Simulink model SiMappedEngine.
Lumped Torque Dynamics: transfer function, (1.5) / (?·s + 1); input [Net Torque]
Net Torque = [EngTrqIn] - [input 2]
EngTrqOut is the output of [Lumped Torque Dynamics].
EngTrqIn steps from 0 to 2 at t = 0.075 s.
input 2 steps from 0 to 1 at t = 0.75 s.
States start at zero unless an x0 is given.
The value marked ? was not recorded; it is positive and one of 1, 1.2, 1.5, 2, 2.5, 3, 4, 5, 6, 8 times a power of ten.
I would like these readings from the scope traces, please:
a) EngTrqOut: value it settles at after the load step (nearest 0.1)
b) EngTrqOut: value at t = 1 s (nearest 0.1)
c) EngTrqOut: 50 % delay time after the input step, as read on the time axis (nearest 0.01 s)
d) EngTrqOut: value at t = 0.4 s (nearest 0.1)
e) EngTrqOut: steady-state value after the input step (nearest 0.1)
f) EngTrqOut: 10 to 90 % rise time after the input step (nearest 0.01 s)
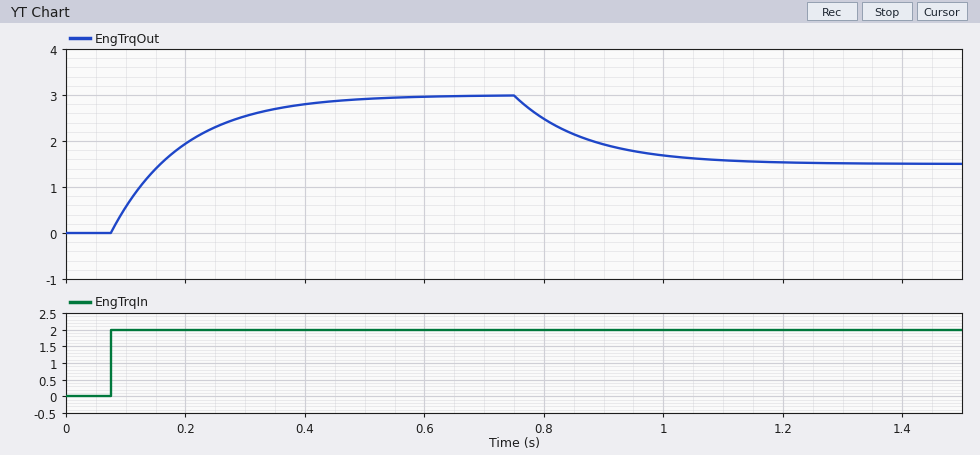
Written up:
1.5
1.7
0.16 s
2.8
3.0
0.26 s
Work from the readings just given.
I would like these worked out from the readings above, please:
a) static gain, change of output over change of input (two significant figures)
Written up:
1.5
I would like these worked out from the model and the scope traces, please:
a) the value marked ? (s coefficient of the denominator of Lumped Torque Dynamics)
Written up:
0.12
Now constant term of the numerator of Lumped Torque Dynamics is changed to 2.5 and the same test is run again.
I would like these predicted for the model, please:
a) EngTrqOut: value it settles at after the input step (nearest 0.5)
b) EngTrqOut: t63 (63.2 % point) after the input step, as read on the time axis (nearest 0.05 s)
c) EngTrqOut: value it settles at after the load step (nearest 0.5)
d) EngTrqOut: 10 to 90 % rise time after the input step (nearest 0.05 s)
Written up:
5.0
0.20 s
2.5
0.25 s
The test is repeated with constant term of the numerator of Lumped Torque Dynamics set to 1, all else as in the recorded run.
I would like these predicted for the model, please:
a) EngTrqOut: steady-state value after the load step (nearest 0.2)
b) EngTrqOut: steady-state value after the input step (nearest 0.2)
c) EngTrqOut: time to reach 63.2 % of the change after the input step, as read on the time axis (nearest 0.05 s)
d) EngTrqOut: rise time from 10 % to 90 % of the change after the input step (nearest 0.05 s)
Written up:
1.0
2.0
0.20 s
0.25 s
